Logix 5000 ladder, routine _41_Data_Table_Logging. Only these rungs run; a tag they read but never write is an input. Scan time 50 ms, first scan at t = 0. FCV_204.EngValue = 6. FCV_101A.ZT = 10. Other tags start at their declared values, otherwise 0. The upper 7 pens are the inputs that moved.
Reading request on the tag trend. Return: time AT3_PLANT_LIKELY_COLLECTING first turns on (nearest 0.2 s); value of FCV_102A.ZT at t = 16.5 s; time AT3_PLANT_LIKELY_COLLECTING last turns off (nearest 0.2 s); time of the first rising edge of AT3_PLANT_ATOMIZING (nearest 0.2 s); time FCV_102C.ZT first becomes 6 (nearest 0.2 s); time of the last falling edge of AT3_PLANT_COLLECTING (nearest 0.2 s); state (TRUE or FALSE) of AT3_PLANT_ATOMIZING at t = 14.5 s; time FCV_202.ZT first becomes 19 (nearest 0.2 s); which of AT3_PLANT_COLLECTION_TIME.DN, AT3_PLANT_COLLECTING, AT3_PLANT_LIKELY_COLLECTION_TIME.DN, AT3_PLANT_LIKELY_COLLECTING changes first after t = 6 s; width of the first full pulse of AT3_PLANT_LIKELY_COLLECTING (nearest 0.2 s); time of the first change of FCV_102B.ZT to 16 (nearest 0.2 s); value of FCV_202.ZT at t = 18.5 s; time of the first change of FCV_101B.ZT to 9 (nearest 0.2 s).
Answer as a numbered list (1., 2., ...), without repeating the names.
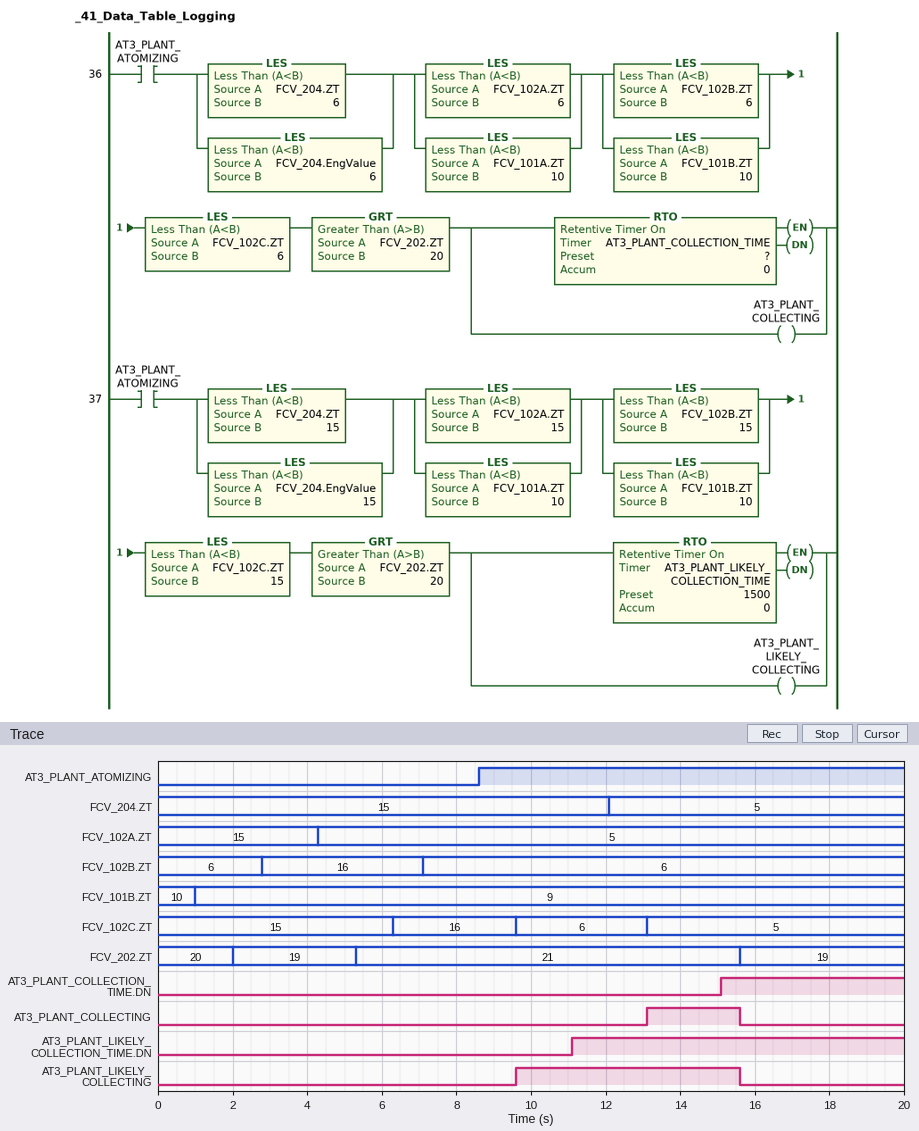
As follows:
1. 9.6 s
2. 5
3. 15.6 s
4. 8.6 s
5. 9.6 s
6. 15.6 s
7. TRUE
8. 2.0 s
9. AT3_PLANT_LIKELY_COLLECTING
10. 6.0 s
11. 2.8 s
12. 19
13. 1.0 s
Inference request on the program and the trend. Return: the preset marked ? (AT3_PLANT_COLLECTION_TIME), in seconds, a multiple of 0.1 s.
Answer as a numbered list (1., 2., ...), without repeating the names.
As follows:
1. 2.0 s
